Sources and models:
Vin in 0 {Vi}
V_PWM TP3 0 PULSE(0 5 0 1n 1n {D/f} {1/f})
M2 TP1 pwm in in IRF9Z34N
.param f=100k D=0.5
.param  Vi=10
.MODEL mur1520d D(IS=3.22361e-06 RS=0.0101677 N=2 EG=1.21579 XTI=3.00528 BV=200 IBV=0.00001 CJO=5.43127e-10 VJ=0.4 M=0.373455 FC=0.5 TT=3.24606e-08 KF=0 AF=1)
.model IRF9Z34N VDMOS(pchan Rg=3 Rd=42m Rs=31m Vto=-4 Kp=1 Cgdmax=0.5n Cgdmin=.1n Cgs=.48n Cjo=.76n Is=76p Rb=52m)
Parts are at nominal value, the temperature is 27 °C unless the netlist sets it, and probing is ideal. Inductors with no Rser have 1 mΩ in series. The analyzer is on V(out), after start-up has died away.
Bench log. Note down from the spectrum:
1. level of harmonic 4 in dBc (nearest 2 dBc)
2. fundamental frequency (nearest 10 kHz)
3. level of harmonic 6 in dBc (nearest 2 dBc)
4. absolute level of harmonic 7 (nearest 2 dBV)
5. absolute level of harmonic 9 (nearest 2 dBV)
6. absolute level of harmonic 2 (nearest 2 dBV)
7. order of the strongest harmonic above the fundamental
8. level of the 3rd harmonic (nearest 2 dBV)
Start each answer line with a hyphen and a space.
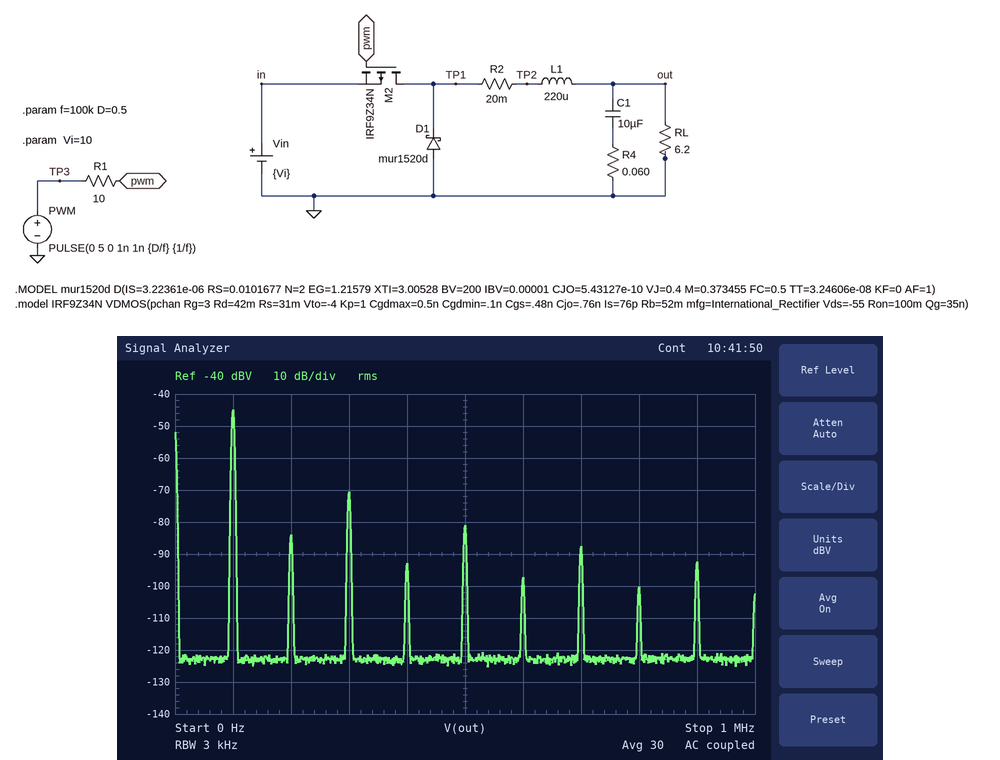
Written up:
- -48 dBc
- 100 kHz
- -52 dBc
- -88 dBV
- -92 dBV
- -84 dBV
- 3
- -70 dBV
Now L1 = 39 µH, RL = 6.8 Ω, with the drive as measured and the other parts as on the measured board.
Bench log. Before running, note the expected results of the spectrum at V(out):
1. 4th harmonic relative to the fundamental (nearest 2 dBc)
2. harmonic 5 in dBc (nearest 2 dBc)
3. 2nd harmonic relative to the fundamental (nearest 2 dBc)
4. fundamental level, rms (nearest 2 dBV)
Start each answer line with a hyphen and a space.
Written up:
- -38 dBc
- -40 dBc
- -28 dBc
- -30 dBV
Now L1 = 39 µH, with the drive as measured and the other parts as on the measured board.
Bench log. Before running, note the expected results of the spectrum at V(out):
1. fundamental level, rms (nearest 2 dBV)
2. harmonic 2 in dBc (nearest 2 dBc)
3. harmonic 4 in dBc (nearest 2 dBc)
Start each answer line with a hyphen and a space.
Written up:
- -30 dBV
- -36 dBc
- -46 dBc
